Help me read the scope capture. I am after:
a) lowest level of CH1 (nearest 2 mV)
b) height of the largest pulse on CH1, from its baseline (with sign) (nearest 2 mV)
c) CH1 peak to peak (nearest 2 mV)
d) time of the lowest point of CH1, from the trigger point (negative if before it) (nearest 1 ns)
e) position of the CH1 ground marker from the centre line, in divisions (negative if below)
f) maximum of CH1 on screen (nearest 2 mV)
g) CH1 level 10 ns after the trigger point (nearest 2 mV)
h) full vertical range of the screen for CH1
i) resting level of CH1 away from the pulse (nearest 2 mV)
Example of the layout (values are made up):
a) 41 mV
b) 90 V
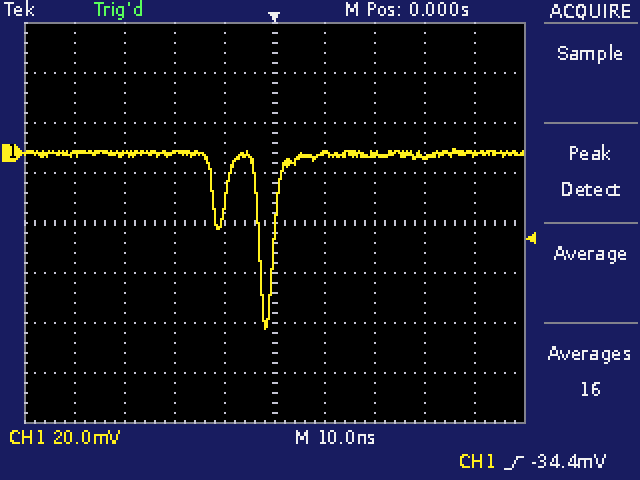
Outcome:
a) -70 mV
b) -70 mV
c) 72 mV
d) -2 ns
e) +1.4 div
f) 2 mV
g) 0 mV
h) 160 mV
i) 0 mV
